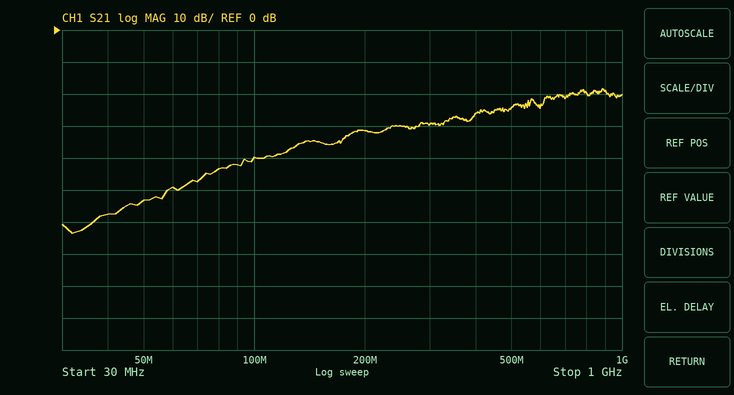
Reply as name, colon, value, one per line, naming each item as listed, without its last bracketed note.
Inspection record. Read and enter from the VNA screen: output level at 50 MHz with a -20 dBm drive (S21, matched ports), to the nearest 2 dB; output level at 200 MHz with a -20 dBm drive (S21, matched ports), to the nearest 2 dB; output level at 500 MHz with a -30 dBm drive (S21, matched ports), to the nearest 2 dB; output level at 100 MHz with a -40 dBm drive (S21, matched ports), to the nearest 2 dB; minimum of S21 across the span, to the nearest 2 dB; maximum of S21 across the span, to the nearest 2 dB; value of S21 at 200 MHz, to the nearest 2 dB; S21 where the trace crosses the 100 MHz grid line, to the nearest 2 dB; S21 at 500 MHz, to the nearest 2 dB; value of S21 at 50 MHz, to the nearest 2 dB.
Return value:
output level at 50 MHz with a -20 dBm drive (S21, matched ports), to the nearest 2 dB: -74 dBm
output level at 200 MHz with a -20 dBm drive (S21, matched ports), to the nearest 2 dB: -52 dBm
output level at 500 MHz with a -30 dBm drive (S21, matched ports), to the nearest 2 dB: -54 dBm
output level at 100 MHz with a -40 dBm drive (S21, matched ports), to the nearest 2 dB: -80 dBm
minimum of S21 across the span, to the nearest 2 dB: -64 dB
maximum of S21 across the span, to the nearest 2 dB: -18 dB
value of S21 at 200 MHz, to the nearest 2 dB: -32 dB
S21 where the trace crosses the 100 MHz grid line, to the nearest 2 dB: -40 dB
S21 at 500 MHz, to the nearest 2 dB: -24 dB
value of S21 at 50 MHz, to the nearest 2 dB: -54 dB
